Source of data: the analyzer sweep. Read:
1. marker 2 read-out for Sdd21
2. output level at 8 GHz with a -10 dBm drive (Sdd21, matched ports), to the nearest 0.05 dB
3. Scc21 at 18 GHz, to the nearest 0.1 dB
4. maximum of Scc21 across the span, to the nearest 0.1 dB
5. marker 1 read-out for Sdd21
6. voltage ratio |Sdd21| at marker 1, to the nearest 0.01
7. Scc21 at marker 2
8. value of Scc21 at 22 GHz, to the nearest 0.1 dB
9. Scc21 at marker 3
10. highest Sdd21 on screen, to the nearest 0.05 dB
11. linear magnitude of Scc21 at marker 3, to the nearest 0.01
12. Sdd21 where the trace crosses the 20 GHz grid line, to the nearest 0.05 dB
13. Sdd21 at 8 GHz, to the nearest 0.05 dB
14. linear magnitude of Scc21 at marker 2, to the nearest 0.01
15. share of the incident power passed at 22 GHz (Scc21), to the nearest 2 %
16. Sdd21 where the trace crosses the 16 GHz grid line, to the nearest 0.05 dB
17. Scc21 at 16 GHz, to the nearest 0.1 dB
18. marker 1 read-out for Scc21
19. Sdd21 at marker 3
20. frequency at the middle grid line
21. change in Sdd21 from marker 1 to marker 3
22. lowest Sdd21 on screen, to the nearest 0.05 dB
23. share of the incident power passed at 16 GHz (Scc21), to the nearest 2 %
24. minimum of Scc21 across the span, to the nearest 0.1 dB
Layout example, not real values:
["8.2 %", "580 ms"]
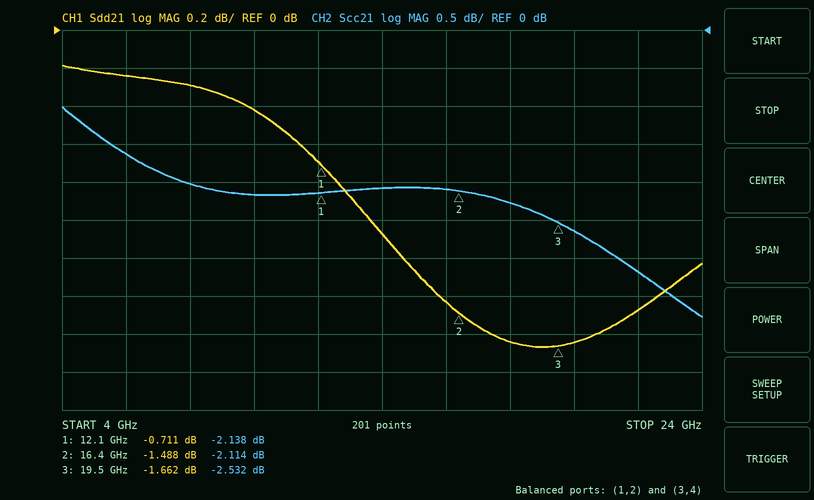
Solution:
["-1.488 dB", "-10.30 dBm", "-2.3 dB", "-1.0 dB", "-0.711 dB", "0.92", "-2.114 dB", "-3.2 dB", "-2.532 dB", "-0.20 dB", "0.75", "-1.65 dB", "-0.30 dB", "0.78", "48 %", "-1.45 dB", "-2.1 dB", "-2.138 dB", "-1.662 dB", "14 GHz", "-0.951 dB", "-1.65 dB", "62 %", "-3.8 dB"]
